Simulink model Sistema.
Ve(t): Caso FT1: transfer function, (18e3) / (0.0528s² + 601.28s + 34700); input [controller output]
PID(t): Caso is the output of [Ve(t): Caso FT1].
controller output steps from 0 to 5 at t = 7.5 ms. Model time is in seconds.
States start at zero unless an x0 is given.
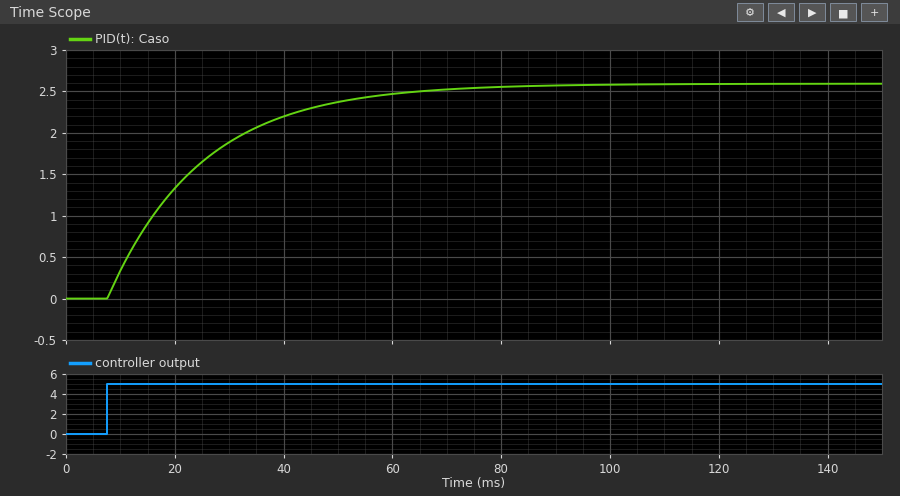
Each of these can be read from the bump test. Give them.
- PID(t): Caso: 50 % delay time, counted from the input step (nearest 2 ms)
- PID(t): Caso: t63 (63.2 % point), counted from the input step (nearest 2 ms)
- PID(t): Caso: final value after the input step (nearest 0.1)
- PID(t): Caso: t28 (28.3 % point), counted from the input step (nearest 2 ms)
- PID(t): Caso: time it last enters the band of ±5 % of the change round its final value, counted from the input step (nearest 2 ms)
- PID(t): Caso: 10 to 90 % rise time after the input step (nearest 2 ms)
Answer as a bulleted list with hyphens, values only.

- 12 ms
- 18 ms
- 2.6
- 6 ms
- 52 ms
- 38 ms
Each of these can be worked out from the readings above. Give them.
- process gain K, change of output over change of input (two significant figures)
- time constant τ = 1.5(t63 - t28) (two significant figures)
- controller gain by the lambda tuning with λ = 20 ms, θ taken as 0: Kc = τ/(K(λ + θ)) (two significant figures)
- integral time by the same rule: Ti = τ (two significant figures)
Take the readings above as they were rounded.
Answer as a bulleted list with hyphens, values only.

- 0.52
- 18 ms
- 1.7
- 18 ms
